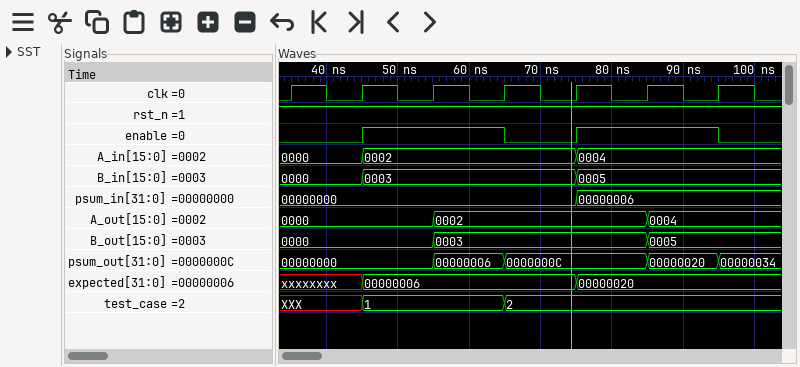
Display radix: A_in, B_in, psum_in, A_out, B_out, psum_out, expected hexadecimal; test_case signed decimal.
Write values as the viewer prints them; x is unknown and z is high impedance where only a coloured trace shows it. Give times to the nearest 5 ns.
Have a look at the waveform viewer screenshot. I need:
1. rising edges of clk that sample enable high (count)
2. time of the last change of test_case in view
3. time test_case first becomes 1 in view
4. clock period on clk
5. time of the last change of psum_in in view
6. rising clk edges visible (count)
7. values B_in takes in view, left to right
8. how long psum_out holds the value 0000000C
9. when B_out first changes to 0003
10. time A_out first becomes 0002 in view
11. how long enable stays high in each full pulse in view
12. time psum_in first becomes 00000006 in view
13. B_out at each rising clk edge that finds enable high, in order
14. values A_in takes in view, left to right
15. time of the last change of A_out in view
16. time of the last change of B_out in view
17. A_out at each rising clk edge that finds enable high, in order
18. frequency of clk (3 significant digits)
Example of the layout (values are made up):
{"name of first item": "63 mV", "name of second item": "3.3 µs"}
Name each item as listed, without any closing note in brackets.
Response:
{"rising edges of clk that sample enable high": "4", "time of the last change of test_case in view": "65 ns", "time test_case first becomes 1 in view": "45 ns", "clock period on clk": "10 ns", "time of the last change of psum_in in view": "75 ns", "rising clk edges visible": "7", "values B_in takes in view, left to right": "0000, 0003, 0005", "how long psum_out holds the value 0000000C": "20 ns", "when B_out first changes to 0003": "55 ns", "time A_out first becomes 0002 in view": "55 ns", "how long enable stays high in each full pulse in view": "20 ns, 20 ns", "time psum_in first becomes 00000006 in view": "75 ns", "B_out at each rising clk edge that finds enable high, in order": "0000, 0003, 0003, 0005", "values A_in takes in view, left to right": "0000, 0002, 0004", "time of the last change of A_out in view": "85 ns", "time of the last change of B_out in view": "85 ns", "A_out at each rising clk edge that finds enable high, in order": "0000, 0002, 0002, 0004", "frequency of clk": "100 MHz"}
